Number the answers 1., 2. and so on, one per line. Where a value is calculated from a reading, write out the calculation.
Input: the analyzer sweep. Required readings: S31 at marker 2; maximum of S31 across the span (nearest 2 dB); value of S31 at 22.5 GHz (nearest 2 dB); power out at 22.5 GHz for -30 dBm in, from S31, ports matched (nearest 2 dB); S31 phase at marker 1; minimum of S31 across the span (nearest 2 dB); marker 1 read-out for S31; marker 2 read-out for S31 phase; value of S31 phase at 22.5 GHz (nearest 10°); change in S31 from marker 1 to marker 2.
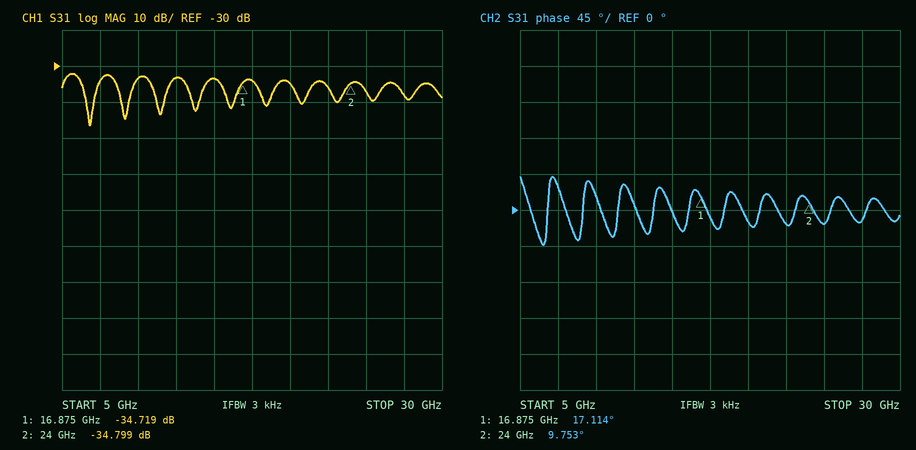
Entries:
1. -34.799 dB
2. -32 dB
3. -36 dB
4. -30 dBm + (-36 dB) = -66 dBm
5. 17.114°
6. -46 dB
7. -34.719 dB
8. 9.753°
9. -20°
10. -34.799 − (-34.719) = -0.080 dB
